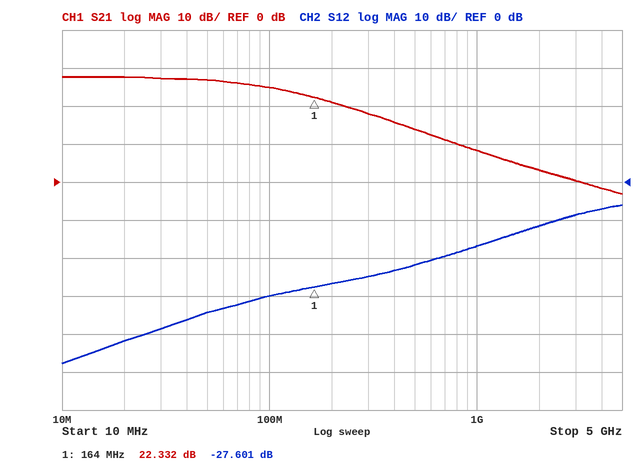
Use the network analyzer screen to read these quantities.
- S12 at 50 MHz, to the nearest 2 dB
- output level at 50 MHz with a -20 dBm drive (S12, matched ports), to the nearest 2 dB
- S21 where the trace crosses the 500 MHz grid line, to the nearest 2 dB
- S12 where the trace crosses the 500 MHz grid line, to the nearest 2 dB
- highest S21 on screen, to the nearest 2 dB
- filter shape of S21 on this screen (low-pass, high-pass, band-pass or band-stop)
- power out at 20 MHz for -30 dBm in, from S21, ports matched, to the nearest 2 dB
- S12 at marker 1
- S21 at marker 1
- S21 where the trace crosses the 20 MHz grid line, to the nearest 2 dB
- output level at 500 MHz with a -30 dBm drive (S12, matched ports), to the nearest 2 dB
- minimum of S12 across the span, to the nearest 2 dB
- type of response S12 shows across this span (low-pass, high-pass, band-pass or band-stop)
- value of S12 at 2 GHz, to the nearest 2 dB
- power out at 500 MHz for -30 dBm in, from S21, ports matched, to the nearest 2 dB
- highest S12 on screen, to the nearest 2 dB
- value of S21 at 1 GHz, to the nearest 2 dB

-34 dB
-54 dBm
14 dB
-22 dB
28 dB
low-pass
-2 dBm
-27.601 dB
22.332 dB
28 dB
-52 dBm
-48 dB
high-pass
-12 dB
-16 dBm
-6 dB
8 dB
